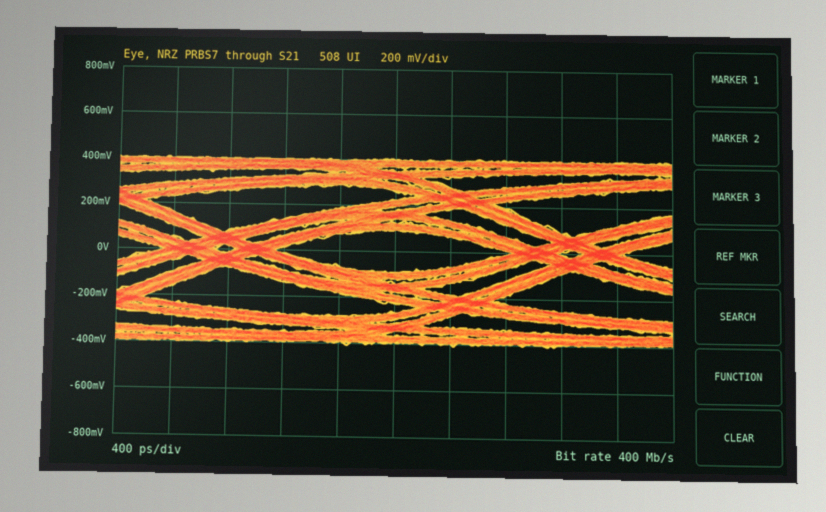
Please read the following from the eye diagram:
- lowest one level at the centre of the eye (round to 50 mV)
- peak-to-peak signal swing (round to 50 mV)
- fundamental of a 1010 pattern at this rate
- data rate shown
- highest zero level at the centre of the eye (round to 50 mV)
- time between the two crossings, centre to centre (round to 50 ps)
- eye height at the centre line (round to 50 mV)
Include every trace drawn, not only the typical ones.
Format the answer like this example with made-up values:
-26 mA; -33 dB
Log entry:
100 mV; 800 mV; 200 MHz; 400 Mb/s; -100 mV; 2.50 ns; 200 mV
